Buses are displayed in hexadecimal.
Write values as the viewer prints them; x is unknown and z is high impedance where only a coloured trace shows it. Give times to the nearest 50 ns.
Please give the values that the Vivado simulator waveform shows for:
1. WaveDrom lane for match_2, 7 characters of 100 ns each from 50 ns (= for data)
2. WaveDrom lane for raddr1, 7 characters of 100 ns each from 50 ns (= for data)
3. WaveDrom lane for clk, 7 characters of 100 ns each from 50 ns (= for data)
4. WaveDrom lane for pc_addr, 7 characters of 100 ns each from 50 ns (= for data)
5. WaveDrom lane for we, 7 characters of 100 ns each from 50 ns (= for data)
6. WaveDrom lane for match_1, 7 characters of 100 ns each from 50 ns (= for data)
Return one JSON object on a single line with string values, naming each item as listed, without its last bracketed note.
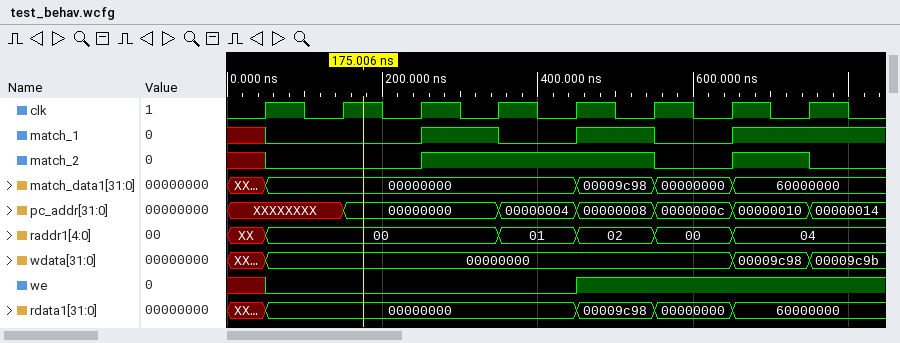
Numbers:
{"WaveDrom lane for match_2, 7 characters of 100 ns each from 50 ns": "{name: 'match_2', wave: '0.1..01'}", "WaveDrom lane for raddr1, 7 characters of 100 ns each from 50 ns": "{name: 'raddr1', wave: '=..====', data: '00 01 02 00 04'}", "WaveDrom lane for clk, 7 characters of 100 ns each from 50 ns": "{name: 'clk', wave: 'p......'}", "WaveDrom lane for pc_addr, 7 characters of 100 ns each from 50 ns": "{name: 'pc_addr', wave: 'x=.====', data: '00000000 00000004 00000008 0000000c 00000010'}", "WaveDrom lane for we, 7 characters of 100 ns each from 50 ns": "{name: 'we', wave: '0...1..'}", "WaveDrom lane for match_1, 7 characters of 100 ns each from 50 ns": "{name: 'match_1', wave: '0.10101'}"}
